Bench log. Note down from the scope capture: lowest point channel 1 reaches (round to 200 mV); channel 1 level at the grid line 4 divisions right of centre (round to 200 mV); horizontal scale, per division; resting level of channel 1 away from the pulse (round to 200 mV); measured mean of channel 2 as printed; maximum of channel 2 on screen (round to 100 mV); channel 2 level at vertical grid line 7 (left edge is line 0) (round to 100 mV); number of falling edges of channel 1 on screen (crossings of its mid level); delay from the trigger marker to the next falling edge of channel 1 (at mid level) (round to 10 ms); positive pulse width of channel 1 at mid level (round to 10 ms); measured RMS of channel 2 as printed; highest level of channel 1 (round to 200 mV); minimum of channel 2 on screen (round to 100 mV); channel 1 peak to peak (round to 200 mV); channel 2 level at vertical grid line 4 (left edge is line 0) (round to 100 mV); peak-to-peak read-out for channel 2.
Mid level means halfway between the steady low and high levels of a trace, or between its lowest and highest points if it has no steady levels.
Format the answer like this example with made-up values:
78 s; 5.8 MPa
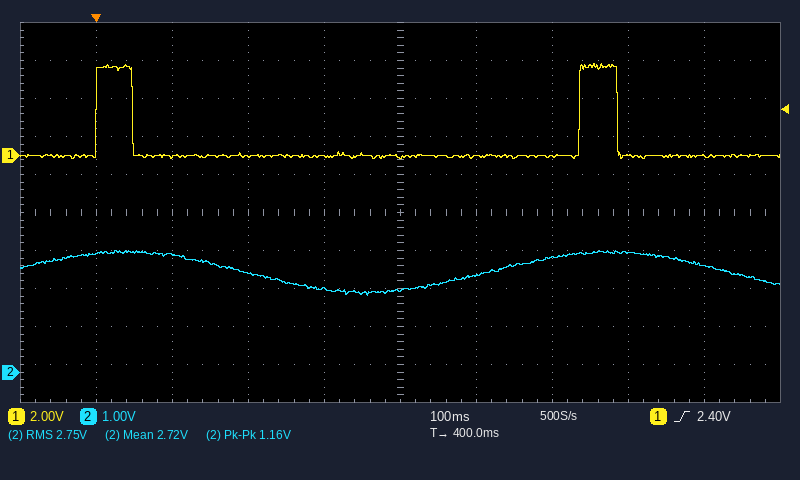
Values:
-200 mV; 0.0 V; 100 ms; 0.0 V; 2.72 V; 3.2 V; 3.0 V; 2; 50 ms; 50 ms; 2.75 V; 4.8 V; 2.0 V; 5.0 V; 2.2 V; 1.16 V
